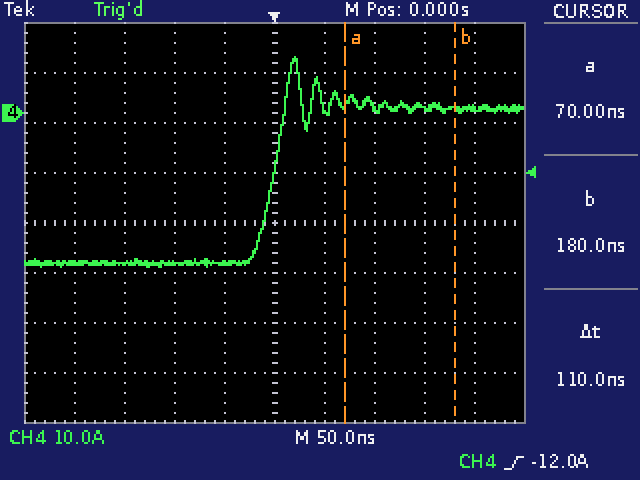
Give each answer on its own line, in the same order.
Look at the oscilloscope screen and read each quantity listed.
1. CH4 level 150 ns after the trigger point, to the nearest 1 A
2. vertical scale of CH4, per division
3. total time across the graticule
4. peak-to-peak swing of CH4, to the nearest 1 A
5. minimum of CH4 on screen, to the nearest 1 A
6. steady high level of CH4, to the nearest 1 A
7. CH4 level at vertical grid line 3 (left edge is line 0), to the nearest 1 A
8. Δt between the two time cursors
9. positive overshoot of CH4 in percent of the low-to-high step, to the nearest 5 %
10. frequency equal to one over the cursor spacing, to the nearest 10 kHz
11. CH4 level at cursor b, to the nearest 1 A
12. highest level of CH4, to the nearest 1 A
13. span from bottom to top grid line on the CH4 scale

1 A
10 A
500 ns
42 A
-31 A
1 A
-30 A
110 ns
35 %
9.09 MHz
1 A
11 A
80 A
